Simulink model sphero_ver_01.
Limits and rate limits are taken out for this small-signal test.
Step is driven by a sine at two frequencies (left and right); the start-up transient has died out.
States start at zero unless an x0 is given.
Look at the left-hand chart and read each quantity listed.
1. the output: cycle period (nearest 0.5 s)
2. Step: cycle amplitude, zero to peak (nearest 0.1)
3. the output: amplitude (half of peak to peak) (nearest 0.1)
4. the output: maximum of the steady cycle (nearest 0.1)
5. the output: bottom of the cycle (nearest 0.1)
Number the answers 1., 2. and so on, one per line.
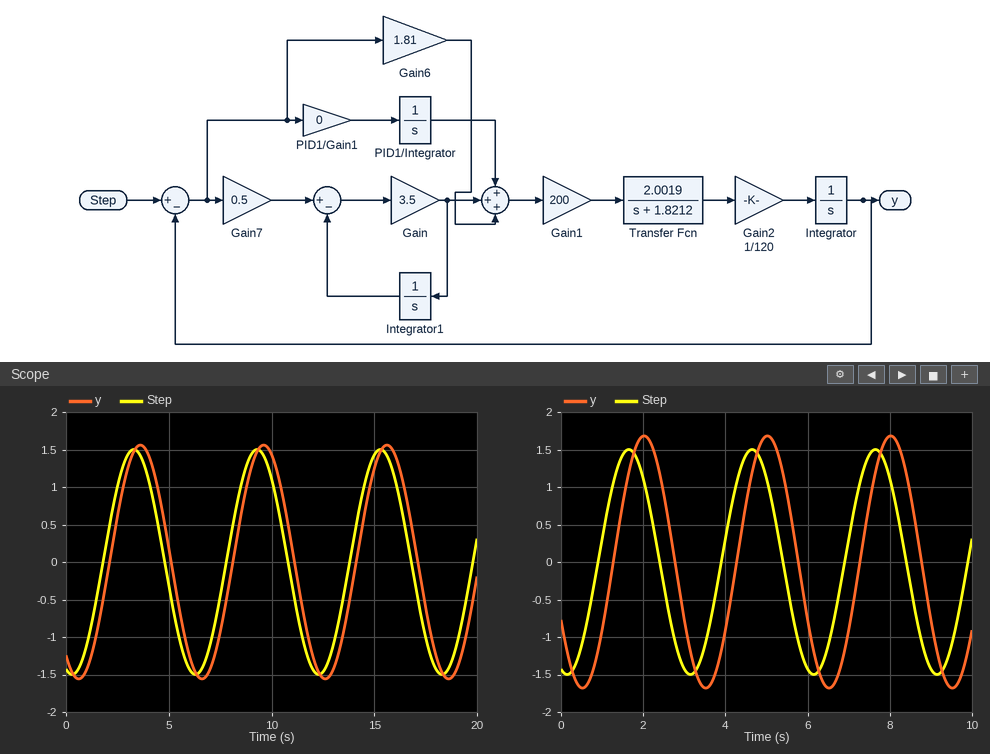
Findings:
1. 6.0 s
2. 1.5
3. 1.6
4. 1.6
5. -1.6
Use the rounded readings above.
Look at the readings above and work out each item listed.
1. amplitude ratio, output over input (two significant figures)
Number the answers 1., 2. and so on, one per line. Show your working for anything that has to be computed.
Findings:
1. 1.6 / 1.5 = 1.1
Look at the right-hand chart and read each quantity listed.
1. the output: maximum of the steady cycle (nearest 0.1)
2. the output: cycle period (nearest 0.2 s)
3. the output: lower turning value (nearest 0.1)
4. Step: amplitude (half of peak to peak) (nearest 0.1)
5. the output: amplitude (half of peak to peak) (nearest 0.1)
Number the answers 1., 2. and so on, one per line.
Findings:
1. 1.7
2. 3.0 s
3. -1.7
4. 1.5
5. 1.7
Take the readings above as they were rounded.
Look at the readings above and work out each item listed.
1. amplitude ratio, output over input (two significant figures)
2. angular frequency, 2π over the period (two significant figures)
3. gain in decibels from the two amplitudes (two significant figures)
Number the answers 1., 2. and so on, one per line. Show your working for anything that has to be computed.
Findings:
1. 1.7 / 1.5 = 1.1
2. 2π / 3 = 2.1 rad/s
3. 20 log10(1.7 / 1.5) = 1.1 dB
